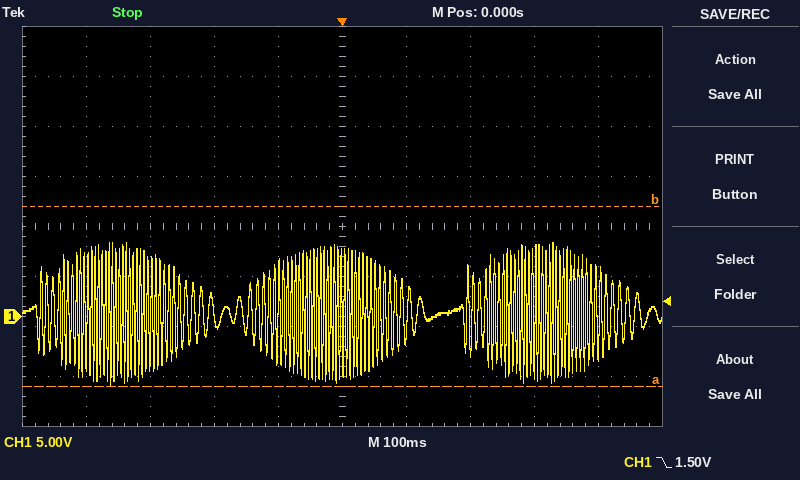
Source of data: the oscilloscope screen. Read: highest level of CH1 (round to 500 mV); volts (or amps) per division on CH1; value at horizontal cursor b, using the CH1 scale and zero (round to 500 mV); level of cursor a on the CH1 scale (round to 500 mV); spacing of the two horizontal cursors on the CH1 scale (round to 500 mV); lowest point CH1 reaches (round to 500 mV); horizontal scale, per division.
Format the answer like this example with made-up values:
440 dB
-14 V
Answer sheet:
7.5 V
5 V
11.0 V
-7.0 V
18.0 V
-7.0 V
100 ms
